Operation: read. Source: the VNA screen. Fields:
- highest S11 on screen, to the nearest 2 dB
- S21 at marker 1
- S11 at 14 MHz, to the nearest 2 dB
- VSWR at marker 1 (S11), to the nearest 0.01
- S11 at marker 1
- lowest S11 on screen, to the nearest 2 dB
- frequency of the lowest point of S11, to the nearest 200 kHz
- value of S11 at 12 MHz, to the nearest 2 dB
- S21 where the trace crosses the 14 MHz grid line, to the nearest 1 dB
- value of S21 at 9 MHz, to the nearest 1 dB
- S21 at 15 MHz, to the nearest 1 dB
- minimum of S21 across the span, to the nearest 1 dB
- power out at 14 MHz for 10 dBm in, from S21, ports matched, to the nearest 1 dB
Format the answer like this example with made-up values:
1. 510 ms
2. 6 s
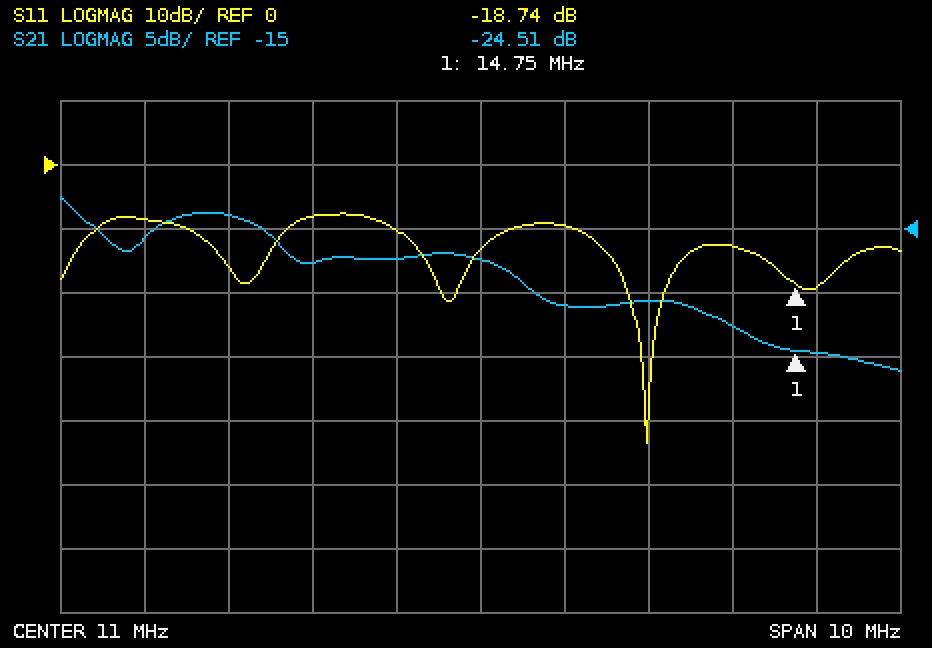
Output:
1. -8 dB
2. -24.51 dB
3. -12 dB
4. 1.26
5. -18.74 dB
6. -44 dB
7. 13.0 MHz
8. -10 dB
9. -23 dB
10. -18 dB
11. -25 dB
12. -26 dB
13. -13 dBm
